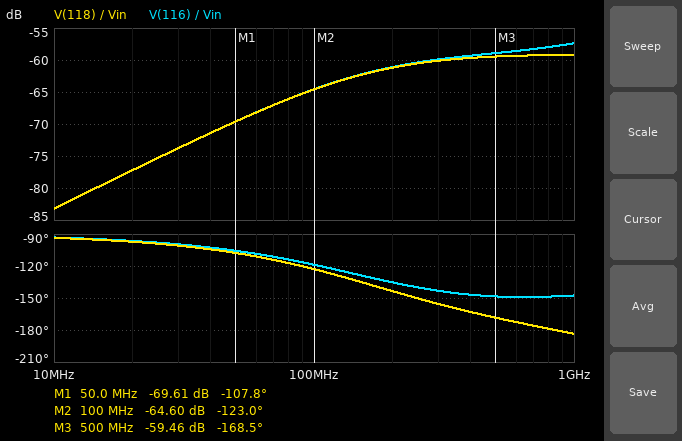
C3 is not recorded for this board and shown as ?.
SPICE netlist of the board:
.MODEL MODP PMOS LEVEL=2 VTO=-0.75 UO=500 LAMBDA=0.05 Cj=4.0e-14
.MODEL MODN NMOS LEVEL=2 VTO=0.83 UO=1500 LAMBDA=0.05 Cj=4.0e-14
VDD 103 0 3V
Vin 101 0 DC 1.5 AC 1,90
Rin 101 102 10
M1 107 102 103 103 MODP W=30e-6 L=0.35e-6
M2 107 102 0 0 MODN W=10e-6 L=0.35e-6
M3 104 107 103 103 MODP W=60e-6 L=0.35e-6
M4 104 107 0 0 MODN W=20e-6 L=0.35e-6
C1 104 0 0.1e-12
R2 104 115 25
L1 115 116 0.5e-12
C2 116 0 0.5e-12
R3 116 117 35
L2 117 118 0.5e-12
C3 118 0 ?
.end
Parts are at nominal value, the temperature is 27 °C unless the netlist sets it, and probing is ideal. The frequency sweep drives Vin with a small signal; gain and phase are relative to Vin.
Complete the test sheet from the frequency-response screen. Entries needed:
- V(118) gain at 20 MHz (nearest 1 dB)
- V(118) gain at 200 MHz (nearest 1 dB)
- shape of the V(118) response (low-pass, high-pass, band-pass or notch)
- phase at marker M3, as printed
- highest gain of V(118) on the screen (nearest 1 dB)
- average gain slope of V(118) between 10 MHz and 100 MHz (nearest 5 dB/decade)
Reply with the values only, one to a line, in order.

-77 dB
-61 dB
high-pass
-168.5 deg
-59 dB
20 dB/decade
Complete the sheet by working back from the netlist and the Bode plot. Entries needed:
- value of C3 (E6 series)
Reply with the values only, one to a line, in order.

3.3 pF
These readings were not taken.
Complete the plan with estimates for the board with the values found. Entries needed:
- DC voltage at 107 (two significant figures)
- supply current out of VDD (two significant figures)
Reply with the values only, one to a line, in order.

2.5 V
380 µA
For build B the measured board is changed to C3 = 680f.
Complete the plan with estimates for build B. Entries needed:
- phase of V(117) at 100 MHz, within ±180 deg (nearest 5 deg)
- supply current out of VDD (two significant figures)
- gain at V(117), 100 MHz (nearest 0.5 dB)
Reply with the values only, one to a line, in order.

-100 deg
380 µA
-63.5 dB
